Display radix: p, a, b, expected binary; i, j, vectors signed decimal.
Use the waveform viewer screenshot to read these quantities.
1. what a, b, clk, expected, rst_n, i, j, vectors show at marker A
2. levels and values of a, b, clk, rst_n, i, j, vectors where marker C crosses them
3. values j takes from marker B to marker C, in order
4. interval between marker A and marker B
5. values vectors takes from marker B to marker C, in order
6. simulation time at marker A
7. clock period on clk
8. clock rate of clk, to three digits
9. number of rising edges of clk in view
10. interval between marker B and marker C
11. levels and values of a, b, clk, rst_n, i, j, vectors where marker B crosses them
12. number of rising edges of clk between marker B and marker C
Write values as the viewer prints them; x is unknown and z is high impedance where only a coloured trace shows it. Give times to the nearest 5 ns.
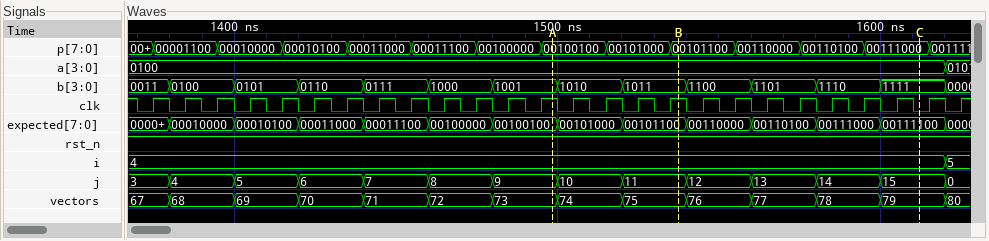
a=0100, b=1001, clk=1, expected=00100100, rst_n=1, i=4, j=9, vectors=73
a=0100, b=1111, clk=0, rst_n=1, i=4, j=15, vectors=79
11, 12, 13, 14, 15
40 ns
75, 76, 77, 78, 79
1500 ns
10 ns
100 MHz
26
75 ns
a=0100, b=1011, clk=1, rst_n=1, i=4, j=11, vectors=75
7
